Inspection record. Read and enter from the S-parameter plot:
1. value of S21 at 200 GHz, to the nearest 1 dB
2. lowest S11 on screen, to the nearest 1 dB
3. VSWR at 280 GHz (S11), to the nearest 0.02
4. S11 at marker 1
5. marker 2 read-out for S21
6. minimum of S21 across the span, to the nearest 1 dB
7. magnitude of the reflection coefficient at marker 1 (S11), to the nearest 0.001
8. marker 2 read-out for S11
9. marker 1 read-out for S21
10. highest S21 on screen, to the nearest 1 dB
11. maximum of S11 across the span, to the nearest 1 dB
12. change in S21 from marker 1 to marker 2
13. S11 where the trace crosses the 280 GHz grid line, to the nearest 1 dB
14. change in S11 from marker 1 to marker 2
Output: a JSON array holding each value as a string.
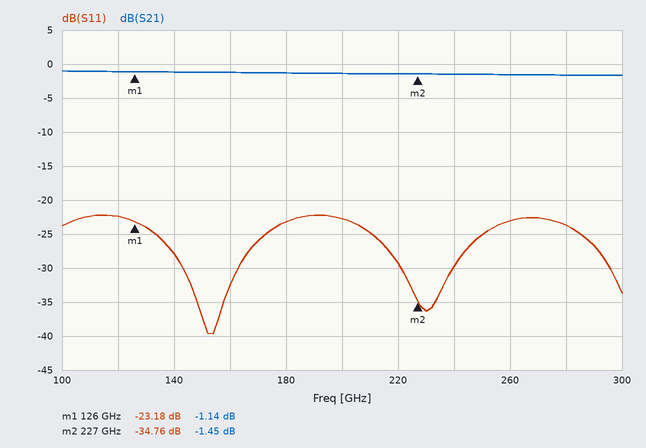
["-1 dB", "-40 dB", "1.14", "-23.18 dB", "-1.45 dB", "-2 dB", "0.069", "-34.76 dB", "-1.14 dB", "-1 dB", "-22 dB", "-0.31 dB", "-24 dB", "-11.58 dB"]
